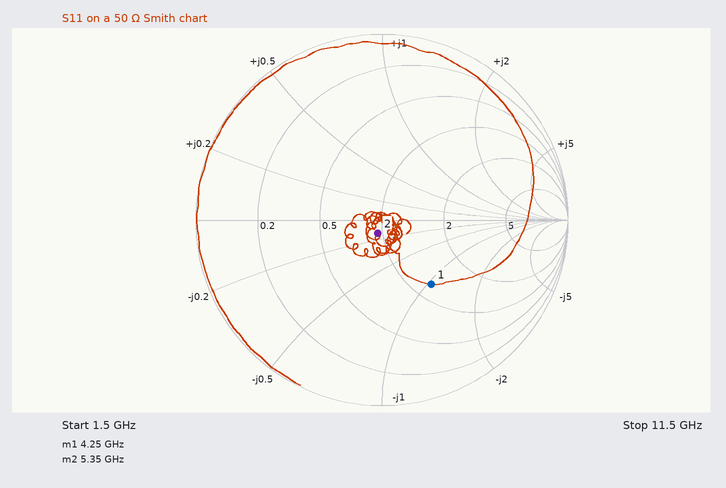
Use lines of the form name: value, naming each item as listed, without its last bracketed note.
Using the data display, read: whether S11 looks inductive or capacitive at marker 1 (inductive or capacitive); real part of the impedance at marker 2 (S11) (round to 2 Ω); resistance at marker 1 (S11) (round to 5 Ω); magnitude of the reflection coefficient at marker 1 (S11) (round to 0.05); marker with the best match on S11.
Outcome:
whether S11 looks inductive or capacitive at marker 1: capacitive
real part of the impedance at marker 2 (S11): 48 Ω
resistance at marker 1 (S11): 60 Ω
magnitude of the reflection coefficient at marker 1 (S11): 0.45
marker with the best match on S11: marker 2
